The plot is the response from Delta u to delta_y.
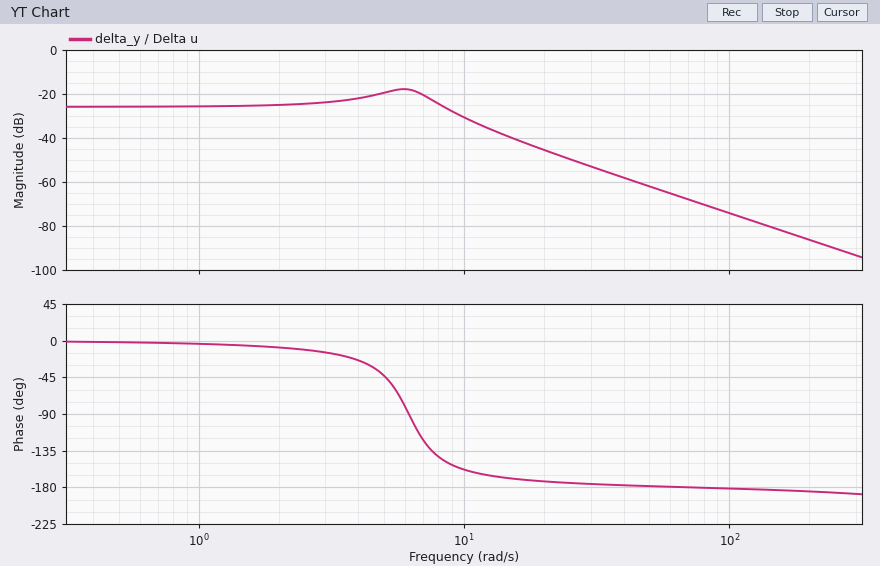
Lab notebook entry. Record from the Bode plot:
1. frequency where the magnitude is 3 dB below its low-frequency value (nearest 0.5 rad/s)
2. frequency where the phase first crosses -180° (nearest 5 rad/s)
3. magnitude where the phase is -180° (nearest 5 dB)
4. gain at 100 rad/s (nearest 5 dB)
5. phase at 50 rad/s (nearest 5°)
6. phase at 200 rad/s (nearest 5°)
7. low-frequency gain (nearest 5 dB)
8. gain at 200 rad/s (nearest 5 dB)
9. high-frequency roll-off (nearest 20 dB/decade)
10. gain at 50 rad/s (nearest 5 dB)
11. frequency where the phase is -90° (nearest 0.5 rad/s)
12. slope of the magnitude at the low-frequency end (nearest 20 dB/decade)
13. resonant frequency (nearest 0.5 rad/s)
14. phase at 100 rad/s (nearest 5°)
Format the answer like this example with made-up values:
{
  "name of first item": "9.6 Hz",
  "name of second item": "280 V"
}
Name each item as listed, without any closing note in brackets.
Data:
{
  "frequency where the magnitude is 3 dB below its low-frequency value": "9.5 rad/s",
  "frequency where the phase first crosses -180°": "70 rad/s",
  "magnitude where the phase is -180°": "-70 dB",
  "gain at 100 rad/s": "-75 dB",
  "phase at 50 rad/s": "-180°",
  "phase at 200 rad/s": "-185°",
  "low-frequency gain": "-25 dB",
  "gain at 200 rad/s": "-85 dB",
  "high-frequency roll-off": "-40 dB/decade",
  "gain at 50 rad/s": "-60 dB",
  "frequency where the phase is -90°": "6.0 rad/s",
  "slope of the magnitude at the low-frequency end": "0 dB/decade",
  "resonant frequency": "6.0 rad/s",
  "phase at 100 rad/s": "-180°"
}
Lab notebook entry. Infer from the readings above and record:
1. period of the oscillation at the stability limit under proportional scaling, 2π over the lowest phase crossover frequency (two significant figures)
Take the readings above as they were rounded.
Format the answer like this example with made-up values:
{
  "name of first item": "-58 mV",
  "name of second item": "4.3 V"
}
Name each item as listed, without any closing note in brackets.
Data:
{
  "period of the oscillation at the stability limit under proportional scaling, 2π over the lowest phase crossover frequency": "0.090 s"
}
